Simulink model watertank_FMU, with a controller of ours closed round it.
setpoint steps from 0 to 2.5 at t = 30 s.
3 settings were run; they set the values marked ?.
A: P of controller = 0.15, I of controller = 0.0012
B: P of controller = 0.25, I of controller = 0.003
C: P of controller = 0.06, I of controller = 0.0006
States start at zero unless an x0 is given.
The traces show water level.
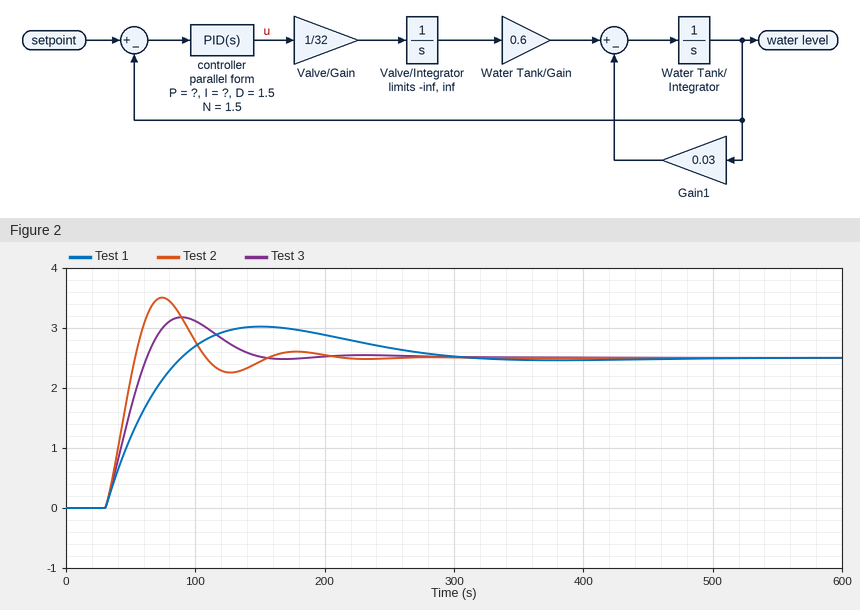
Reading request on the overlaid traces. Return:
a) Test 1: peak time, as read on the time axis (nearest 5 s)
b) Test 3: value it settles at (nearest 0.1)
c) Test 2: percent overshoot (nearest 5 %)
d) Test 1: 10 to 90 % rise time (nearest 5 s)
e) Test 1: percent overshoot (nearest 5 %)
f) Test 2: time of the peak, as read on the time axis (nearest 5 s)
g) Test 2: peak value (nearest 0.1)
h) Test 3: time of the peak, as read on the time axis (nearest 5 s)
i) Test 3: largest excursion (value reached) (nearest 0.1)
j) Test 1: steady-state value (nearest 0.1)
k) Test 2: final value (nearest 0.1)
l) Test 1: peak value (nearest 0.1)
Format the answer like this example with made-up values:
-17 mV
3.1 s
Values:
150 s
2.5
40 %
45 s
20 %
75 s
3.5
90 s
3.2
2.5
2.5
3.0
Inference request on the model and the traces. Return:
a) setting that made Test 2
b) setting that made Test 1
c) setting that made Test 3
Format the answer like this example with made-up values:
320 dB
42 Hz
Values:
B
C
A
